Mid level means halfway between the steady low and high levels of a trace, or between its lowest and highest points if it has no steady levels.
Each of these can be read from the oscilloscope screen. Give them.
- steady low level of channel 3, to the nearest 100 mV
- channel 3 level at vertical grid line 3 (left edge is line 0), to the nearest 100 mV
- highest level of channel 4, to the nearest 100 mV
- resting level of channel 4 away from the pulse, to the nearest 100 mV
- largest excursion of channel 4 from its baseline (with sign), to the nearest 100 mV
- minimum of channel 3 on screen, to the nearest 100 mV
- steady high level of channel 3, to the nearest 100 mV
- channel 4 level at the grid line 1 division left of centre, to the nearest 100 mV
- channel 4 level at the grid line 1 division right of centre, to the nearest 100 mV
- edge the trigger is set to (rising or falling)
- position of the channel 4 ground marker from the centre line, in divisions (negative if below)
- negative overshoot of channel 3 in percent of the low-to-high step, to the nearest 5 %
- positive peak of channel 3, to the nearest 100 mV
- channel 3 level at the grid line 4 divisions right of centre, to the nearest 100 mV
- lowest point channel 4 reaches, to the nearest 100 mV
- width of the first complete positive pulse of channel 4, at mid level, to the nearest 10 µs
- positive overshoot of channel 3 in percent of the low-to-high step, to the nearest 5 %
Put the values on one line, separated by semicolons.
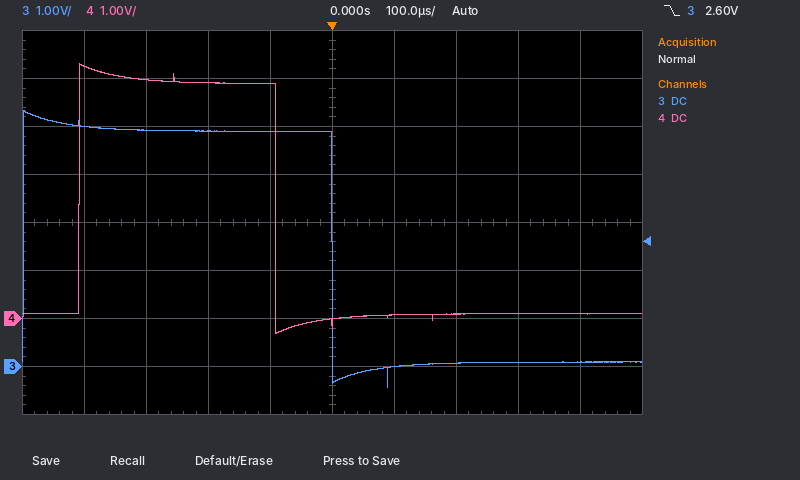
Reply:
100 mV; 4.9 V; 5.3 V; 100 mV; +5.2 V; -400 mV; 4.9 V; 4.9 V; 100 mV; falling; -2.0 div; 10 %; 5.3 V; 100 mV; -300 mV; 320 µs; 10 %
